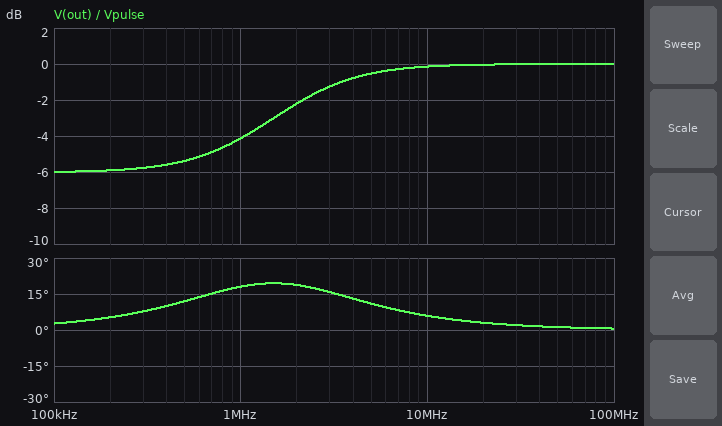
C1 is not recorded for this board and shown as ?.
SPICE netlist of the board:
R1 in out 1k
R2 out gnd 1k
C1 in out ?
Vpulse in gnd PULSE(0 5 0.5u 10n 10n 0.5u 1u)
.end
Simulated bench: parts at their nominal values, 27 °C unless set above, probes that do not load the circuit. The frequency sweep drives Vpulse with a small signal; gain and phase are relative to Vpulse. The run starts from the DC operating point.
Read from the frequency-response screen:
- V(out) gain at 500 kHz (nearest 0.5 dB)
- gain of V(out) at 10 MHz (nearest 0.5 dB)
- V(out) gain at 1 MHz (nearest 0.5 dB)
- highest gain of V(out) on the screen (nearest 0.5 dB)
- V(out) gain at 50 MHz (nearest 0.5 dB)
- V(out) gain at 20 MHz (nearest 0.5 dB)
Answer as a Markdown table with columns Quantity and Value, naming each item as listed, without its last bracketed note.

| Quantity | Value |
|---|---|
| V(out) gain at 500 kHz | -5.5 dB |
| gain of V(out) at 10 MHz | 0 dB |
| V(out) gain at 1 MHz | -4.0 dB |
| highest gain of V(out) on the screen | 0 dB |
| V(out) gain at 50 MHz | 0 dB |
| V(out) gain at 20 MHz | 0 dB |
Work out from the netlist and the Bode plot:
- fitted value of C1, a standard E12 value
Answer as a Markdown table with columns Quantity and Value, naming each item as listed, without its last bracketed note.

| Quantity | Value |
|---|---|
| fitted value of C1, a standard E12 value | 150 pF |
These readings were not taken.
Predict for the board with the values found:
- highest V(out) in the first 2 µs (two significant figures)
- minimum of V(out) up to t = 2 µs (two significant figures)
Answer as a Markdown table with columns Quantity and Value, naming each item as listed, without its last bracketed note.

| Quantity | Value |
|---|---|
| highest V(out) in the first 2 µs | 4.8 V |
| minimum of V(out) up to t = 2 µs | -2.3 V |
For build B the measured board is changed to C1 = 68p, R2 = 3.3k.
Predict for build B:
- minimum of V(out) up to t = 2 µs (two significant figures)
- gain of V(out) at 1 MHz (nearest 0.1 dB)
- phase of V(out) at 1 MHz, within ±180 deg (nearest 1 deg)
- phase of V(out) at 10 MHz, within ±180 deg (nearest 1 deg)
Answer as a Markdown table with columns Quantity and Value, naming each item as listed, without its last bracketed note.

| Quantity | Value |
|---|---|
| minimum of V(out) up to t = 2 µs | -1.1 V |
| gain of V(out) at 1 MHz | -2.0 dB |
| phase of V(out) at 1 MHz, within ±180 deg | 5 deg |
| phase of V(out) at 10 MHz, within ±180 deg | 4 deg |
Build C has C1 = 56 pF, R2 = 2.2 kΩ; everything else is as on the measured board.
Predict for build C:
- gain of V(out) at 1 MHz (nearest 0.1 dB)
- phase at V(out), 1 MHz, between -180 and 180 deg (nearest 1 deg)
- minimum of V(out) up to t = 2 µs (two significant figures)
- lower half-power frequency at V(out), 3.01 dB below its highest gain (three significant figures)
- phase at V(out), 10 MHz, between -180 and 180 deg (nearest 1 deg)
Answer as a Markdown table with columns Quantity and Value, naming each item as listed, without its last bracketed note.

| Quantity | Value |
|---|---|
| gain of V(out) at 1 MHz | -3.0 dB |
| phase at V(out), 1 MHz, between -180 and 180 deg | 6 deg |
| minimum of V(out) up to t = 2 µs | -1.4 V |
| lower half-power frequency at V(out), 3.01 dB below its highest gain | 967 kHz |
| phase at V(out), 10 MHz, between -180 and 180 deg | 7 deg |
